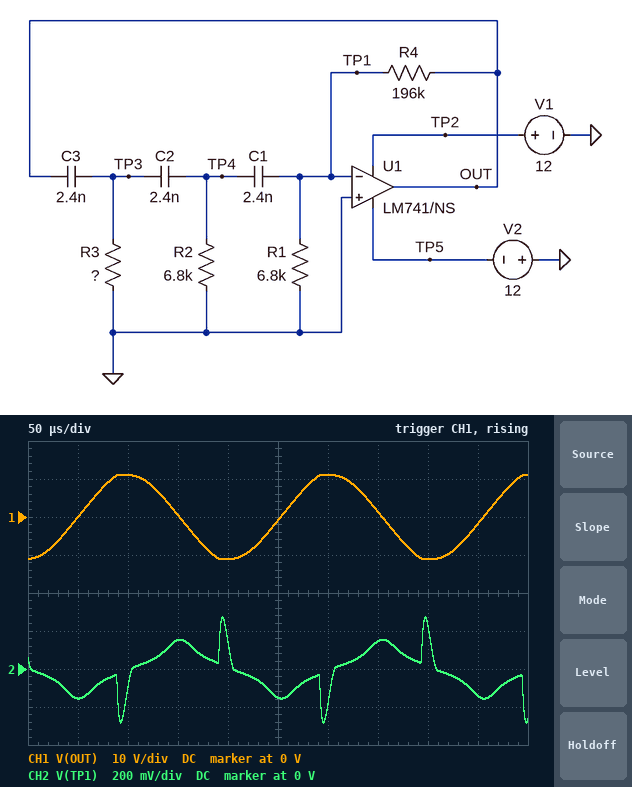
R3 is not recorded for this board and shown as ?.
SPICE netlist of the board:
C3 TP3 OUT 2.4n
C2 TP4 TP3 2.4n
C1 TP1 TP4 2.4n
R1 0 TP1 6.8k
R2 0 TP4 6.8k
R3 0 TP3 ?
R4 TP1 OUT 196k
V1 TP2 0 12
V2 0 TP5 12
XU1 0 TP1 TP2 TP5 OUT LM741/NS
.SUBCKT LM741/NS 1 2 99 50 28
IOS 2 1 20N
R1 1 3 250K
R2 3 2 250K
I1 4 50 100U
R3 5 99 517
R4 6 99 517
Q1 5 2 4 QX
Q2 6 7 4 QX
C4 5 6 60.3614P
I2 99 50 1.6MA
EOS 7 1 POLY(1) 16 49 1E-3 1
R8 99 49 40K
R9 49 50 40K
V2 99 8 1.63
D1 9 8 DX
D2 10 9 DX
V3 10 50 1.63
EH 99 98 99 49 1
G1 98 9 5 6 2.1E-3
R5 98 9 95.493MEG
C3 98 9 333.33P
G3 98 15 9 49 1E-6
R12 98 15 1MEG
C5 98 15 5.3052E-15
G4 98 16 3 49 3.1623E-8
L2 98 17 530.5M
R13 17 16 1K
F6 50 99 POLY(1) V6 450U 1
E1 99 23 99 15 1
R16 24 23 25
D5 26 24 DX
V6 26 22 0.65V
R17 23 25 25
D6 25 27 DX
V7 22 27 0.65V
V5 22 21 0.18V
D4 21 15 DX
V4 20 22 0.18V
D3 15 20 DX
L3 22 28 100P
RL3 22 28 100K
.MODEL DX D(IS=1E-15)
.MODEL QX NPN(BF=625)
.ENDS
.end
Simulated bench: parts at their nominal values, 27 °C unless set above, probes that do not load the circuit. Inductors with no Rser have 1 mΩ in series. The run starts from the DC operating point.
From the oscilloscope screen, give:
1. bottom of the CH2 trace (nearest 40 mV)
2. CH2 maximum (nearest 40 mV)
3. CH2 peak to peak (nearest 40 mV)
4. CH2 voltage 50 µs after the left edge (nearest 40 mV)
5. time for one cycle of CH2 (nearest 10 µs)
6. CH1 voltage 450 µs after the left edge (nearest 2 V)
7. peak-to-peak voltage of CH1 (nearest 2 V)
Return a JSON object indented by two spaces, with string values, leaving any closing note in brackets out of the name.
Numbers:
{
  "bottom of the CH2 trace": "-280 mV",
  "CH2 maximum": "280 mV",
  "CH2 peak to peak": "560 mV",
  "CH2 voltage 50 µs after the left edge": "-160 mV",
  "time for one cycle of CH2": "200 µs",
  "CH1 voltage 450 µs after the left edge": "-2 V",
  "peak-to-peak voltage of CH1": "22 V"
}
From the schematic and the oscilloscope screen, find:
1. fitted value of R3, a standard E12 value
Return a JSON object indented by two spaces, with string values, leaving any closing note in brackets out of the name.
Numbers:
{
  "fitted value of R3, a standard E12 value": "3.3 kΩ"
}
